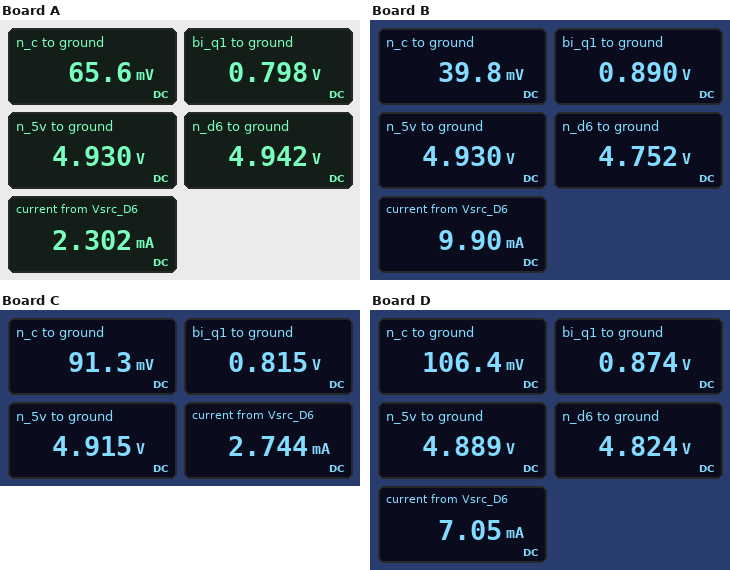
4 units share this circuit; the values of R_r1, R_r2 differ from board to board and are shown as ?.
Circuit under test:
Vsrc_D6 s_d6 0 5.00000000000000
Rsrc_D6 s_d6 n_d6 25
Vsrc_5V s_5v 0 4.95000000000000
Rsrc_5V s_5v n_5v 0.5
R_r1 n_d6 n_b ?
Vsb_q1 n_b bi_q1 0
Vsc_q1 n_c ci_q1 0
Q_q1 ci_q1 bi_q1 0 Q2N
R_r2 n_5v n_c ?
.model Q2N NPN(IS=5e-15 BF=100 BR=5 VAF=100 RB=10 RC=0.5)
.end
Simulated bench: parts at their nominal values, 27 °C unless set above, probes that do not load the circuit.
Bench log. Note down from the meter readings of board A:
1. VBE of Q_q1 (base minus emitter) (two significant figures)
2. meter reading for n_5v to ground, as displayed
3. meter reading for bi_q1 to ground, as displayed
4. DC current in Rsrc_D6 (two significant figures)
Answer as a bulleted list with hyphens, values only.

- 800 mV
- 4.930 V
- 0.798 V
- 2.3 mA
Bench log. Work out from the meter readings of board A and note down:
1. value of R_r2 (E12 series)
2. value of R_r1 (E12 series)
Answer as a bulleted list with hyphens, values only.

- 120 Ω
- 1.8 kΩ
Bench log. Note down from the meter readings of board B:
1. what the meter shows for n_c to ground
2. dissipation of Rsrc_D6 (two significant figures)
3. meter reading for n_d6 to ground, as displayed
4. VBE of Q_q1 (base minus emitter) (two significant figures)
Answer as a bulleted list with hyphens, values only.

- 39.8 mV
- 2.5 mW
- 4.752 V
- 890 mV
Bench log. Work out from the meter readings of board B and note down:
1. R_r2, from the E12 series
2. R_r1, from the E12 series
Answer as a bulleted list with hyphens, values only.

- 120 Ω
- 390 Ω
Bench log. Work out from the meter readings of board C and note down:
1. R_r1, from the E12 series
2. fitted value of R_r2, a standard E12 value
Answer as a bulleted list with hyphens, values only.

- 1.5 kΩ
- 68 Ω
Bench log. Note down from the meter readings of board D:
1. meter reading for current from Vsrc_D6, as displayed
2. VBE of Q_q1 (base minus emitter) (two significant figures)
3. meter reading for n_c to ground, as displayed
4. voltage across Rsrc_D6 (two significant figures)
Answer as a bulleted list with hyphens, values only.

- 7.05 mA
- 870 mV
- 106.4 mV
- 180 mV
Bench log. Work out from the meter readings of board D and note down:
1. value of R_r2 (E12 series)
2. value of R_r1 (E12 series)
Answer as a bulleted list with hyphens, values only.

- 39 Ω
- 560 Ω
